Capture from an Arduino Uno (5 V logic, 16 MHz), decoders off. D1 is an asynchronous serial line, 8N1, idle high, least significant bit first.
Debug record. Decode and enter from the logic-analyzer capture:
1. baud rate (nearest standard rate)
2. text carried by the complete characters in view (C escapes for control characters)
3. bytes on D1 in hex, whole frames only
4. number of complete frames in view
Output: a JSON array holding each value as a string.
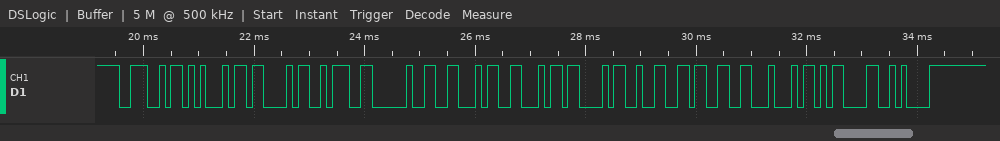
["9600 baud", "\"NEC: FFC23D\\r\\n\"", "4E 45 43 3A 20 46 46 43 32 33 44 0D 0A", "13"]
